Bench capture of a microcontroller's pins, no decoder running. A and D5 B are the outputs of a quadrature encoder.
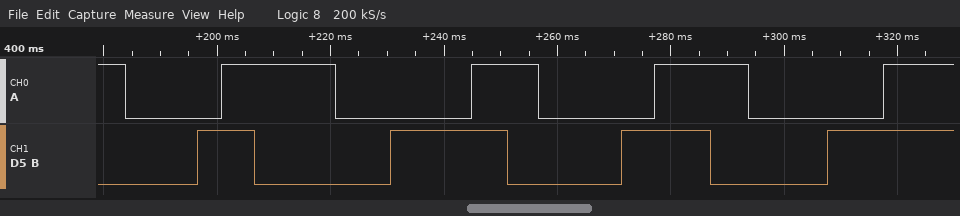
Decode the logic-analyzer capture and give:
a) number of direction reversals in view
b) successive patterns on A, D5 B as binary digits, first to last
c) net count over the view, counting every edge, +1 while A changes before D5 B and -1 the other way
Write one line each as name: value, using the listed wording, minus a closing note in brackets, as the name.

number of direction reversals in view: 0
successive patterns on A, D5 B as binary digits, first to last: 10 00 01 11 10 00 01 11 10 00 01 11 10 00 01 11
net count over the view, counting every edge, +1 while A changes before D5 B and -1 the other way: -15
